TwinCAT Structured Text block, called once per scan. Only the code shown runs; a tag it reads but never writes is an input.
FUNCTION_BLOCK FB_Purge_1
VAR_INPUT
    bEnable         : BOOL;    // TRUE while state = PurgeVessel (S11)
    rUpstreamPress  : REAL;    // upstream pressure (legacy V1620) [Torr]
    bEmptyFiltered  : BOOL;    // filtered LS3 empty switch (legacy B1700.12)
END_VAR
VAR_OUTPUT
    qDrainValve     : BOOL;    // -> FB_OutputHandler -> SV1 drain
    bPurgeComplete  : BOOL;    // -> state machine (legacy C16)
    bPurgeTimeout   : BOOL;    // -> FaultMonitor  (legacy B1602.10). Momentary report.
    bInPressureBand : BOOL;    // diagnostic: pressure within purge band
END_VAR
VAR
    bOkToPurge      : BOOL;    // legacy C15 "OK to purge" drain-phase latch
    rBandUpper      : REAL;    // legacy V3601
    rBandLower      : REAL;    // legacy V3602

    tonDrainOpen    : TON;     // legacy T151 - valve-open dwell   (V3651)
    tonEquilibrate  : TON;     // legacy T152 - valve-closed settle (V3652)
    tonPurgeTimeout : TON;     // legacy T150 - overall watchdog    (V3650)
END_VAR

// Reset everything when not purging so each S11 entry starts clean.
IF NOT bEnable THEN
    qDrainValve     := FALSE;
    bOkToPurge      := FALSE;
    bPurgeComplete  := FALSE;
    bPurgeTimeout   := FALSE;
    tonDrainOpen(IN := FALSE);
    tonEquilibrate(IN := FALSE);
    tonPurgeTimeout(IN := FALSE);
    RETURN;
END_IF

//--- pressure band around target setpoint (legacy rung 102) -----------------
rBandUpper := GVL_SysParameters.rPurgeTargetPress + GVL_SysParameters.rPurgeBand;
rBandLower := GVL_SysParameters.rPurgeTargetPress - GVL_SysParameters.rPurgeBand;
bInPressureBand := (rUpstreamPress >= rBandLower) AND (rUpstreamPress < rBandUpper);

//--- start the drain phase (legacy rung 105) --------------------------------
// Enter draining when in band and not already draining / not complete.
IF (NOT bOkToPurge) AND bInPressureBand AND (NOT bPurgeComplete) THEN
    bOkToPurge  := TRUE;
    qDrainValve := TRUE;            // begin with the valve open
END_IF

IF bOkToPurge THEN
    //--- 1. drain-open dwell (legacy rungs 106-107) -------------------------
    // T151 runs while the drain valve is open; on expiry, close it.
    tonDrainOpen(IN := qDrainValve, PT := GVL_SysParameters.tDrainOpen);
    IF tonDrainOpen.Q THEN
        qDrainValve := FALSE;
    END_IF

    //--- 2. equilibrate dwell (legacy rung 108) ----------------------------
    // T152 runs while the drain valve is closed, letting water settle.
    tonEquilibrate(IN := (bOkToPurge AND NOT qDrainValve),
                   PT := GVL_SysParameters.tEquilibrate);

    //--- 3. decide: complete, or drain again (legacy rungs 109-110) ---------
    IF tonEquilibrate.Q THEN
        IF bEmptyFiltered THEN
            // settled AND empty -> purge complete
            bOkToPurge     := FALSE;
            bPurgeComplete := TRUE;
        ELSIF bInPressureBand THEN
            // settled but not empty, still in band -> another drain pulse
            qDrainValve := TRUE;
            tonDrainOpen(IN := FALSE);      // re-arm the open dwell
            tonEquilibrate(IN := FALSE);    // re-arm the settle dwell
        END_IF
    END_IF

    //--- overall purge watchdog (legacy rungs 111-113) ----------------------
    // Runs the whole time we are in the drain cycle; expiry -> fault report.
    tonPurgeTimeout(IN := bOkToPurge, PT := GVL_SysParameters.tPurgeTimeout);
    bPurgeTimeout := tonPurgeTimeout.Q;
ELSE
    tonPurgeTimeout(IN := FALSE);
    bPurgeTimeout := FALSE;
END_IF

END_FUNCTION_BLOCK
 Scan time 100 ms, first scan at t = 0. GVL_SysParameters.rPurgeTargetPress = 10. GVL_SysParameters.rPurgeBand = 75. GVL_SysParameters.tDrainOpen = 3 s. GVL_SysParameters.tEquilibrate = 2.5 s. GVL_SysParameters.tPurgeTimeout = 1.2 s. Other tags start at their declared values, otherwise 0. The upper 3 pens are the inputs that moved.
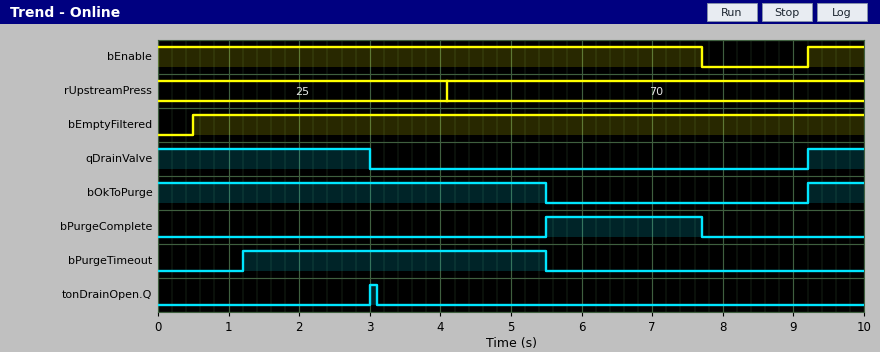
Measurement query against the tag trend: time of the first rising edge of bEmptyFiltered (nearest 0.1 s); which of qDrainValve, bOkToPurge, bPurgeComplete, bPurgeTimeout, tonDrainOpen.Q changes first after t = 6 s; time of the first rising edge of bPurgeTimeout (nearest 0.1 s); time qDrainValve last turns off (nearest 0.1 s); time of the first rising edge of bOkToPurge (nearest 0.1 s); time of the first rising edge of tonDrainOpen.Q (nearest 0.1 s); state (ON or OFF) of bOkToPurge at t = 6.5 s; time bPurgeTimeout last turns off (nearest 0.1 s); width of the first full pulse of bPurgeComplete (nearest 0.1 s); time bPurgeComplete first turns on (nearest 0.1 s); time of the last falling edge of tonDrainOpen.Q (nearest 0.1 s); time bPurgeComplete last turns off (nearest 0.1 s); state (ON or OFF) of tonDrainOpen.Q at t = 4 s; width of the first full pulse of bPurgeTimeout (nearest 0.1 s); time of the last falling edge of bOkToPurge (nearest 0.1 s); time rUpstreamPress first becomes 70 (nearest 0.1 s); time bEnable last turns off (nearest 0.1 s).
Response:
0.5 s
bPurgeComplete
1.2 s
3.0 s
9.2 s
3.0 s
OFF
5.5 s
2.2 s
5.5 s
3.1 s
7.7 s
OFF
4.3 s
5.5 s
4.1 s
7.7 s
